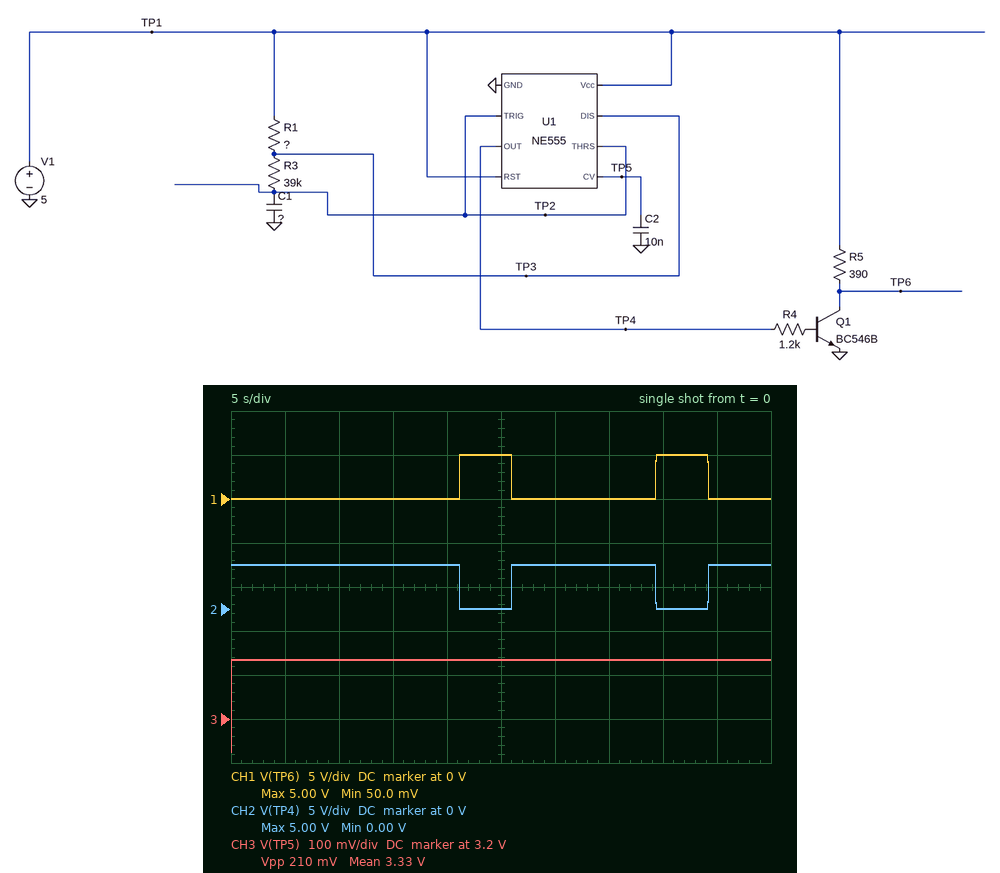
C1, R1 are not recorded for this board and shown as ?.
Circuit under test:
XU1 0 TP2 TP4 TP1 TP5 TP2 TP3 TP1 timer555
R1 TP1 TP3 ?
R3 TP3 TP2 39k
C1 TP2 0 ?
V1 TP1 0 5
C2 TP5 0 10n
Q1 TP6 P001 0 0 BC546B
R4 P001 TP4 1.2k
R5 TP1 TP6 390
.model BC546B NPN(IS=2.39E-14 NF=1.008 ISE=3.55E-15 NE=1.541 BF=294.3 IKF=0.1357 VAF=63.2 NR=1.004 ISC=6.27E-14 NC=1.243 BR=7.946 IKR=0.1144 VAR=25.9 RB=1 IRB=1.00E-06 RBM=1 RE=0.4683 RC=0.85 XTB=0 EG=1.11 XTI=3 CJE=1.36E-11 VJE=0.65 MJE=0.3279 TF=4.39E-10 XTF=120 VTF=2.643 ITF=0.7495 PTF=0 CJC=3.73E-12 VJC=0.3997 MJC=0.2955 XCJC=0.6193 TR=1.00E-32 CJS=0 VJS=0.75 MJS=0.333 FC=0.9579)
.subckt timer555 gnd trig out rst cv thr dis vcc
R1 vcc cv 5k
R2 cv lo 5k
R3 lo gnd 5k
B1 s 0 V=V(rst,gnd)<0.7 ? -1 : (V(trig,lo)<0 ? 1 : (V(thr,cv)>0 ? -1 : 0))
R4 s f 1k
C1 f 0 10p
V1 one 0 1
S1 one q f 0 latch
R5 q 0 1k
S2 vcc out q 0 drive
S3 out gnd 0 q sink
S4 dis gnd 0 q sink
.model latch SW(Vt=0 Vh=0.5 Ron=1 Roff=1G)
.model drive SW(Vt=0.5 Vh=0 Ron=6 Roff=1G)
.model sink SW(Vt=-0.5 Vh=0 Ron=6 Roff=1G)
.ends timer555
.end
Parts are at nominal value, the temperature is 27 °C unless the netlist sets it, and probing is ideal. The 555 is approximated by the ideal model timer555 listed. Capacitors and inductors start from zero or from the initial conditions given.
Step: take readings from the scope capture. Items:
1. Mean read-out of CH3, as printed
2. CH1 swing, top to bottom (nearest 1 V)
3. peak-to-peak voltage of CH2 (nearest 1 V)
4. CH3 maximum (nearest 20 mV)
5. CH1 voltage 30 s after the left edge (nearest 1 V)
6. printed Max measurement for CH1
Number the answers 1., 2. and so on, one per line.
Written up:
1. 3.33 V
2. 5 V
3. 5 V
4. 3.34 V
5. 0 V
6. 5.00 V
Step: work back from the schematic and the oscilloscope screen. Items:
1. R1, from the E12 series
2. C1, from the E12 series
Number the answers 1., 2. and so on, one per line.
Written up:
1. 68 kΩ
2. 180 µF
